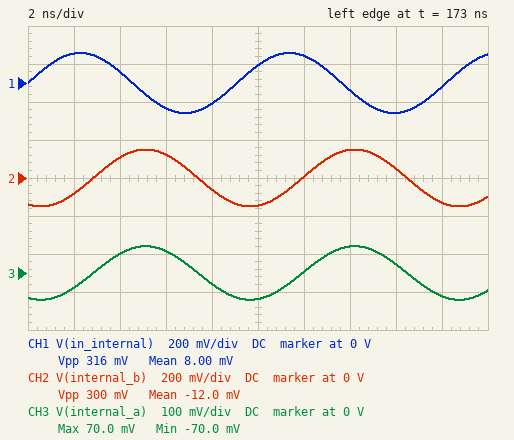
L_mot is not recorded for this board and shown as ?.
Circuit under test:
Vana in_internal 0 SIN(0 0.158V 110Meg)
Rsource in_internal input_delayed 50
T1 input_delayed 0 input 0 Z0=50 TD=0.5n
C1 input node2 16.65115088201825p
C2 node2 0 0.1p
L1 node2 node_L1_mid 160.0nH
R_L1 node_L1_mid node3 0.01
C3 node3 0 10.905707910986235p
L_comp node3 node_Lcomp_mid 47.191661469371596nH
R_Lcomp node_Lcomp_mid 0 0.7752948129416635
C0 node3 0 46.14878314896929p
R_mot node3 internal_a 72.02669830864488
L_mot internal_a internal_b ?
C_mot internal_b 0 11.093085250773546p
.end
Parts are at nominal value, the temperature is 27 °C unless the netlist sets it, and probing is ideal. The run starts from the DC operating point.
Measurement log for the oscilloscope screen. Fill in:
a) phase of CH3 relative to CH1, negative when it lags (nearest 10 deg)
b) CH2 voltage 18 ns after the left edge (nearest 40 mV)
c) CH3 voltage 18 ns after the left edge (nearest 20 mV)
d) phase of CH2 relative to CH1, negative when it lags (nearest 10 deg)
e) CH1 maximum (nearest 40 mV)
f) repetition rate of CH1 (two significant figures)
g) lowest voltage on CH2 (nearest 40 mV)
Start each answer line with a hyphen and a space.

- -110 deg
- -120 mV
- -60 mV
- -110 deg
- 160 mV
- 110 MHz
- -160 mV
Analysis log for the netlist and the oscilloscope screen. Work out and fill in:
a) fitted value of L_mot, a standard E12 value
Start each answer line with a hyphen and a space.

- 100 nH
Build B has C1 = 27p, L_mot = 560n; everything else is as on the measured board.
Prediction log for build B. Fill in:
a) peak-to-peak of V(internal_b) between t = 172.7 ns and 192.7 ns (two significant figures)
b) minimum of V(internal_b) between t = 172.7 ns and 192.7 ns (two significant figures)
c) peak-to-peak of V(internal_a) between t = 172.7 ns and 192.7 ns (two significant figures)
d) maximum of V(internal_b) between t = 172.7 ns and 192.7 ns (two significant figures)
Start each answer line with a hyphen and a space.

- 180 mV
- -89 mV
- 350 mV
- 89 mV
